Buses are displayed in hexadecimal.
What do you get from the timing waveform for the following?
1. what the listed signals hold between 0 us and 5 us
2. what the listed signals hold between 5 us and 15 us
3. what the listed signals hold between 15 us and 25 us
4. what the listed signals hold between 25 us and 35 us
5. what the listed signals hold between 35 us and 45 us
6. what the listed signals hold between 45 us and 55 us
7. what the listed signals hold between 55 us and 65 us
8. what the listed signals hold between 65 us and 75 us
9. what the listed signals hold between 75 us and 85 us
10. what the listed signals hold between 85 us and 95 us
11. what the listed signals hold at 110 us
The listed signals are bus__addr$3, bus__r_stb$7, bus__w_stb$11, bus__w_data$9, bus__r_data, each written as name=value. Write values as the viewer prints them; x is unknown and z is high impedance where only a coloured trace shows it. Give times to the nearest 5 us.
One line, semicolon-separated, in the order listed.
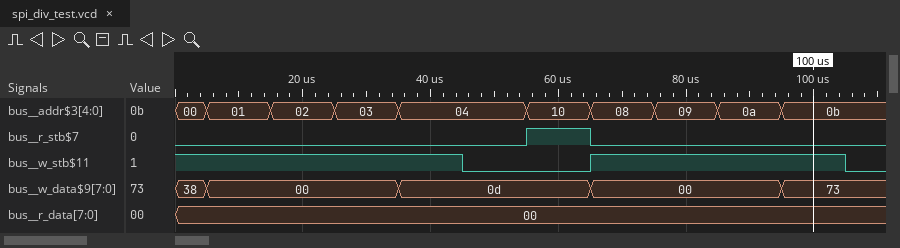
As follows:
bus__addr$3=00, bus__r_stb$7=0, bus__w_stb$11=1, bus__w_data$9=38, bus__r_data=00; bus__addr$3=01, bus__r_stb$7=0, bus__w_stb$11=1, bus__w_data$9=00, bus__r_data=00; bus__addr$3=02, bus__r_stb$7=0, bus__w_stb$11=1, bus__w_data$9=00, bus__r_data=00; bus__addr$3=03, bus__r_stb$7=0, bus__w_stb$11=1, bus__w_data$9=00, bus__r_data=00; bus__addr$3=04, bus__r_stb$7=0, bus__w_stb$11=1, bus__w_data$9=0d, bus__r_data=00; bus__addr$3=04, bus__r_stb$7=0, bus__w_stb$11=0, bus__w_data$9=0d, bus__r_data=00; bus__addr$3=10, bus__r_stb$7=1, bus__w_stb$11=0, bus__w_data$9=0d, bus__r_data=00; bus__addr$3=08, bus__r_stb$7=0, bus__w_stb$11=1, bus__w_data$9=00, bus__r_data=00; bus__addr$3=09, bus__r_stb$7=0, bus__w_stb$11=1, bus__w_data$9=00, bus__r_data=00; bus__addr$3=0a, bus__r_stb$7=0, bus__w_stb$11=1, bus__w_data$9=00, bus__r_data=00; bus__addr$3=0b, bus__r_stb$7=0, bus__w_stb$11=0, bus__w_data$9=73, bus__r_data=00
